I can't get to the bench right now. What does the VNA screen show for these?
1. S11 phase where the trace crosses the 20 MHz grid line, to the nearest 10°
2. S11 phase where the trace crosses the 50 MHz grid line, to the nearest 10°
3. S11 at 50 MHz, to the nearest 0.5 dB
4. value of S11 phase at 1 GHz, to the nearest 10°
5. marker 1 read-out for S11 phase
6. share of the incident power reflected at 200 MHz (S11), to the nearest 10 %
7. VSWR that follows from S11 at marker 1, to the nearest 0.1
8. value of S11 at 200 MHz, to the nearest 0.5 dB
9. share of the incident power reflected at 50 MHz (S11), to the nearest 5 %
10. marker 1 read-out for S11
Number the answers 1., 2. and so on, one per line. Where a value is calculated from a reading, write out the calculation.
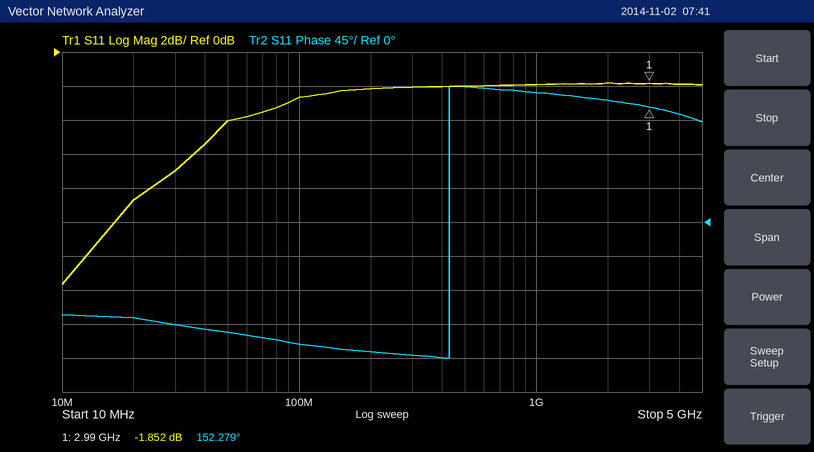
1. -130°
2. -150°
3. -4.0 dB
4. 170°
5. 152.279°
6. 10^(-2/10) ≈ 63.1 %, so 60 % to the nearest 10 %
7. (1 + 0.8080)/(1 − 0.8080) ≈ 9.4
8. -2.0 dB
9. 10^(-4/10) ≈ 40 %
10. -1.852 dB
